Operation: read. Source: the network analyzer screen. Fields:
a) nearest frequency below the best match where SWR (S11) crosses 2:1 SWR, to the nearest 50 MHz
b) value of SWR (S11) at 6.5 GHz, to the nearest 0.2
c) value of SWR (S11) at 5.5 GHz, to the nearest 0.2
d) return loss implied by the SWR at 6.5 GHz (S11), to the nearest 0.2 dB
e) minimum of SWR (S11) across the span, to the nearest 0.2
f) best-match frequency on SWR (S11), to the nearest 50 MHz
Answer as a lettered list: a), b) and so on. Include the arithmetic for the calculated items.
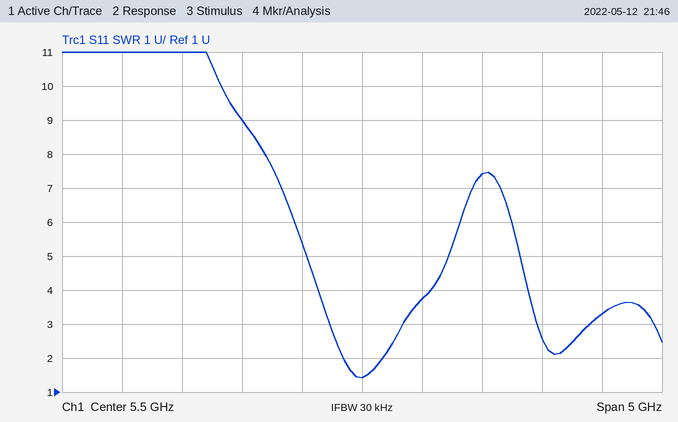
a) 5.35 GHz
b) 7.4
c) 1.4
d) −20 log10((7.4 − 1)/(7.4 + 1)) ≈ 2.4 dB
e) 1.4
f) 5.50 GHz
